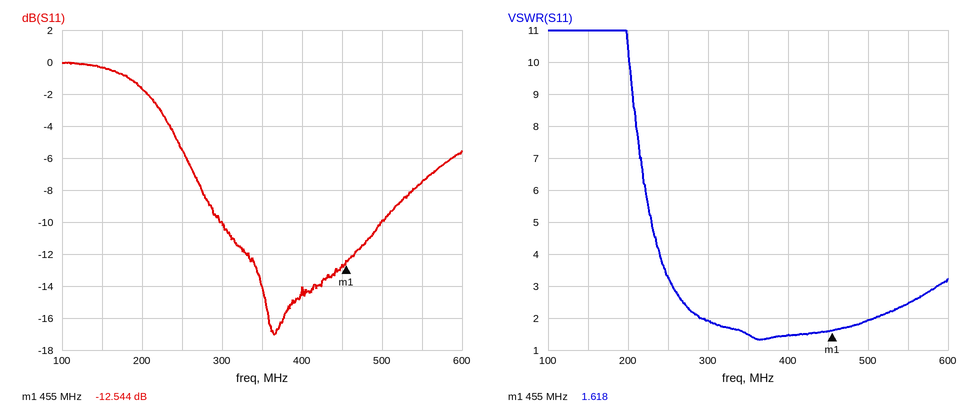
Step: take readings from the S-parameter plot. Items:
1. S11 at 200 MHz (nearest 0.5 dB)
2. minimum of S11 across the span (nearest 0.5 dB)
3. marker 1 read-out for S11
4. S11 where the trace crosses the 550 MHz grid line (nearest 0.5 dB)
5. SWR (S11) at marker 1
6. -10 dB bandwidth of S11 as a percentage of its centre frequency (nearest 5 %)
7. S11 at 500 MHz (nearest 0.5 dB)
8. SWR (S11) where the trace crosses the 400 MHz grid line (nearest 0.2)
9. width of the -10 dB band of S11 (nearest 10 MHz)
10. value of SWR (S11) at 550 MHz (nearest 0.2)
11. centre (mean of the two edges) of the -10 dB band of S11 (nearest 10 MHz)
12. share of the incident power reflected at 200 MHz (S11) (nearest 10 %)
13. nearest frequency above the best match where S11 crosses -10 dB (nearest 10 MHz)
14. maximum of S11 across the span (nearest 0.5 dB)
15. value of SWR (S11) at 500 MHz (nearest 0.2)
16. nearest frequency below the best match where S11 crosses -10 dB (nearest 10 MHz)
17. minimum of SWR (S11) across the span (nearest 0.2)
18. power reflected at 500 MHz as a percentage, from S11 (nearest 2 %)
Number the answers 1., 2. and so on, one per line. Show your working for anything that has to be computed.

1. -1.5 dB
2. -17.0 dB
3. -12.544 dB
4. -7.5 dB
5. 1.618
6. 200 MHz / 400 MHz ≈ 50 %
7. -10.0 dB
8. 1.4
9. 500 MHz − 300 MHz = 200 MHz
10. 2.4
11. 400 MHz
12. 10^(-1.5/10) ≈ 70.8 %, so 70 % to the nearest 10 %
13. 500 MHz
14. 0.0 dB
15. 2.0
16. 300 MHz
17. 1.4
18. 10^(-10/10) ≈ 10 %
